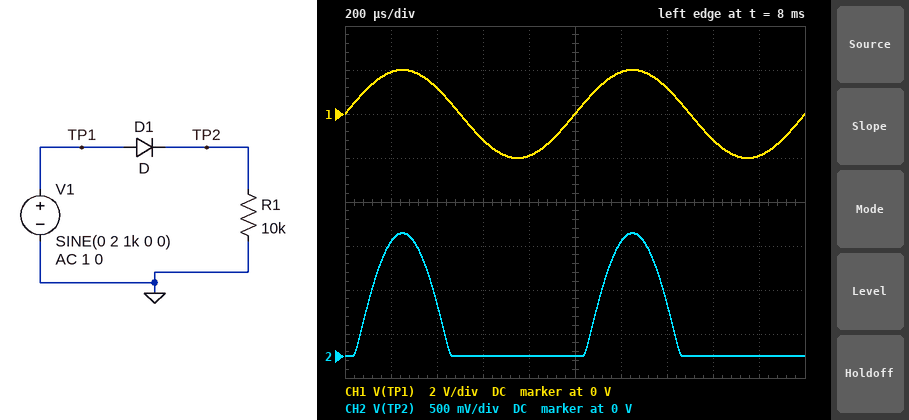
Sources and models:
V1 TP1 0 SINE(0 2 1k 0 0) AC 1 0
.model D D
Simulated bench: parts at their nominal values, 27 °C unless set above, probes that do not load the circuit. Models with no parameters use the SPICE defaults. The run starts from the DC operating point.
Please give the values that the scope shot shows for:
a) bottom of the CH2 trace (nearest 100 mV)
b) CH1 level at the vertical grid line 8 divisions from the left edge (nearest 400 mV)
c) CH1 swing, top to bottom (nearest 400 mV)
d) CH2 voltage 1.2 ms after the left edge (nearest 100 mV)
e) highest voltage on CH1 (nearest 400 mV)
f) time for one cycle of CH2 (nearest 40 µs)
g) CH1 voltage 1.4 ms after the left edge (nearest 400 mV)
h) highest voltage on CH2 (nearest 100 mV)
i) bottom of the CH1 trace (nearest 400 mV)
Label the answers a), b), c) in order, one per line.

a) 0 V
b) -1.2 V
c) 4.0 V
d) 1.3 V
e) 2.0 V
f) 1.00 ms
g) 1.2 V
h) 1.4 V
i) -2.0 V
